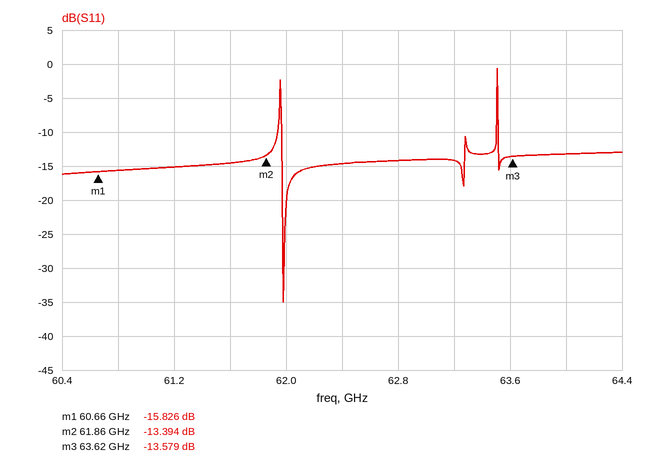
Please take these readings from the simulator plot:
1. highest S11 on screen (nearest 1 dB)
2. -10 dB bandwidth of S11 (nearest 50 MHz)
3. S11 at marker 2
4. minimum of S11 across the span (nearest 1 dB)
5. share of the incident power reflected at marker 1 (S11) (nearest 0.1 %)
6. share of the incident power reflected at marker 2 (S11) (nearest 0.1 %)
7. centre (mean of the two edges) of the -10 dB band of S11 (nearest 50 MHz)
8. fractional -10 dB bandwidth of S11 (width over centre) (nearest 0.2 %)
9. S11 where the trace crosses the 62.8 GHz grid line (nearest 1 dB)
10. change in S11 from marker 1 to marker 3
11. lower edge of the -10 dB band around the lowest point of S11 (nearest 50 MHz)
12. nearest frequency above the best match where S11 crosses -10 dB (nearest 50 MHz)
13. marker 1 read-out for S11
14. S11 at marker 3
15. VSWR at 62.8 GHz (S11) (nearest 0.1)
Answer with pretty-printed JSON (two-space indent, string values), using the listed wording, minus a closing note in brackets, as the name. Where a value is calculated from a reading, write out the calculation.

{
  "highest S11 on screen": "-1 dB",
  "-10 dB bandwidth of S11": "63.50 GHz − 61.95 GHz = 1.55 GHz",
  "S11 at marker 2": "-13.394 dB",
  "minimum of S11 across the span": "-35 dB",
  "share of the incident power reflected at marker 1 (S11)": "10^(-15.826/10) ≈ 2.6 %",
  "share of the incident power reflected at marker 2 (S11)": "10^(-13.394/10) ≈ 4.6 %",
  "centre (mean of the two edges) of the -10 dB band of S11": "62.75 GHz",
  "fractional -10 dB bandwidth of S11 (width over centre)": "1.55 GHz / 62.725 GHz ≈ 2.47 %, so 2.4 % to the nearest 0.2 %",
  "S11 where the trace crosses the 62.8 GHz grid line": "-14 dB",
  "change in S11 from marker 1 to marker 3": "-13.579 − (-15.826) = 2.247 dB",
  "lower edge of the -10 dB band around the lowest point of S11": "61.95 GHz",
  "nearest frequency above the best match where S11 crosses -10 dB": "63.50 GHz",
  "marker 1 read-out for S11": "-15.826 dB",
  "S11 at marker 3": "-13.579 dB",
  "VSWR at 62.8 GHz (S11)": "|Γ| = 10^(-14/20) = 0.1995; VSWR = (1 + 0.1995)/(1 − 0.1995) ≈ 1.5"
}
